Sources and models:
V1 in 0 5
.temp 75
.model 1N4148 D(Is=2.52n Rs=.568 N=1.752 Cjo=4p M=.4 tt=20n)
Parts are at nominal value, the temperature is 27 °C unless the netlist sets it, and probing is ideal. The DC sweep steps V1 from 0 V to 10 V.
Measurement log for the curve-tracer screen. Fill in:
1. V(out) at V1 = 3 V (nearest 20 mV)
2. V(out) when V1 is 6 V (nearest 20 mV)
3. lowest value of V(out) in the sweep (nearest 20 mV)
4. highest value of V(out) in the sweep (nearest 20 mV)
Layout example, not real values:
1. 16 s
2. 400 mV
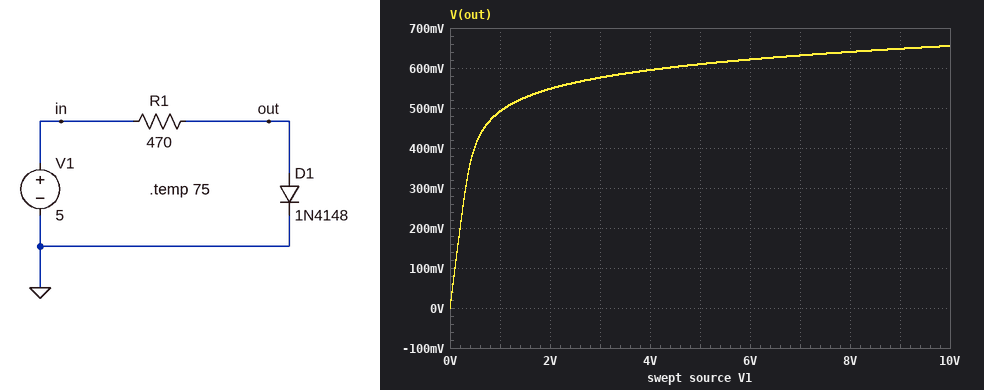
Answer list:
1. 580 mV
2. 620 mV
3. 0 V
4. 660 mV
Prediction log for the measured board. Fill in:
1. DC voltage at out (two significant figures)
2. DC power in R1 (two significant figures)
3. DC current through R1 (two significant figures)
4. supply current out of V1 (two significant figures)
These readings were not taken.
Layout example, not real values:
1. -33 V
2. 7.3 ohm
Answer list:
1. 610 mV
2. 41 mW
3. 9.3 mA
4. 9.3 mA
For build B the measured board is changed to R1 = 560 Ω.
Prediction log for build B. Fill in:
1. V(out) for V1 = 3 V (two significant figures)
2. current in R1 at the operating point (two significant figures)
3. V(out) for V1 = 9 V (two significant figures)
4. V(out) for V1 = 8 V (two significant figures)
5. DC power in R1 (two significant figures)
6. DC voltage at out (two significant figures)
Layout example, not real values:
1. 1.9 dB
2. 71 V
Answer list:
1. 570 mV
2. 7.9 mA
3. 640 mV
4. 630 mV
5. 35 mW
6. 600 mV
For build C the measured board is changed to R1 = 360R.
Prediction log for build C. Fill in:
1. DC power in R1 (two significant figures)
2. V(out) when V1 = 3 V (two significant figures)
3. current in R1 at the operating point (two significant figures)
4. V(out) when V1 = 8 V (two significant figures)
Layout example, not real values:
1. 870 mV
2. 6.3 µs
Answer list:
1. 53 mW
2. 590 mV
3. 12 mA
4. 660 mV
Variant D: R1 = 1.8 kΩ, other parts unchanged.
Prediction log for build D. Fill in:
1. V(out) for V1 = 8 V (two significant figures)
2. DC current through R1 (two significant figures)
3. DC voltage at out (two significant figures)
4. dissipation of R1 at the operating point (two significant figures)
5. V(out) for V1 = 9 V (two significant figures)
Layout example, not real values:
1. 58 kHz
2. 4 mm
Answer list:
1. 560 mV
2. 2.5 mA
3. 540 mV
4. 11 mW
5. 570 mV
